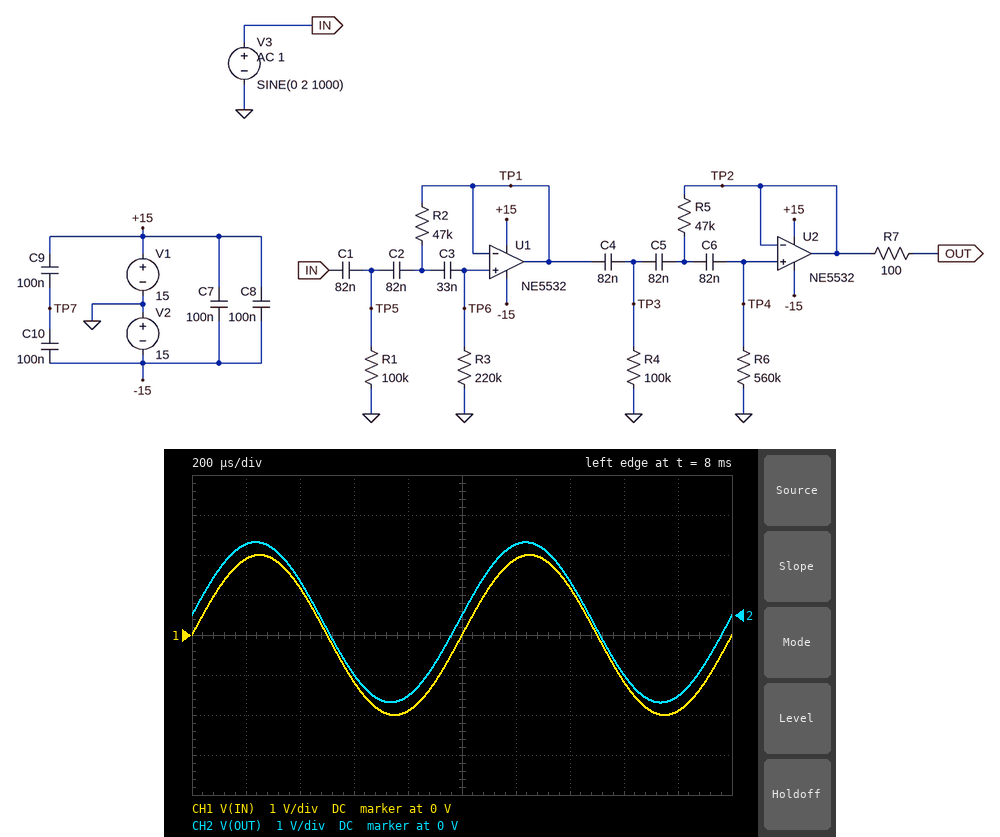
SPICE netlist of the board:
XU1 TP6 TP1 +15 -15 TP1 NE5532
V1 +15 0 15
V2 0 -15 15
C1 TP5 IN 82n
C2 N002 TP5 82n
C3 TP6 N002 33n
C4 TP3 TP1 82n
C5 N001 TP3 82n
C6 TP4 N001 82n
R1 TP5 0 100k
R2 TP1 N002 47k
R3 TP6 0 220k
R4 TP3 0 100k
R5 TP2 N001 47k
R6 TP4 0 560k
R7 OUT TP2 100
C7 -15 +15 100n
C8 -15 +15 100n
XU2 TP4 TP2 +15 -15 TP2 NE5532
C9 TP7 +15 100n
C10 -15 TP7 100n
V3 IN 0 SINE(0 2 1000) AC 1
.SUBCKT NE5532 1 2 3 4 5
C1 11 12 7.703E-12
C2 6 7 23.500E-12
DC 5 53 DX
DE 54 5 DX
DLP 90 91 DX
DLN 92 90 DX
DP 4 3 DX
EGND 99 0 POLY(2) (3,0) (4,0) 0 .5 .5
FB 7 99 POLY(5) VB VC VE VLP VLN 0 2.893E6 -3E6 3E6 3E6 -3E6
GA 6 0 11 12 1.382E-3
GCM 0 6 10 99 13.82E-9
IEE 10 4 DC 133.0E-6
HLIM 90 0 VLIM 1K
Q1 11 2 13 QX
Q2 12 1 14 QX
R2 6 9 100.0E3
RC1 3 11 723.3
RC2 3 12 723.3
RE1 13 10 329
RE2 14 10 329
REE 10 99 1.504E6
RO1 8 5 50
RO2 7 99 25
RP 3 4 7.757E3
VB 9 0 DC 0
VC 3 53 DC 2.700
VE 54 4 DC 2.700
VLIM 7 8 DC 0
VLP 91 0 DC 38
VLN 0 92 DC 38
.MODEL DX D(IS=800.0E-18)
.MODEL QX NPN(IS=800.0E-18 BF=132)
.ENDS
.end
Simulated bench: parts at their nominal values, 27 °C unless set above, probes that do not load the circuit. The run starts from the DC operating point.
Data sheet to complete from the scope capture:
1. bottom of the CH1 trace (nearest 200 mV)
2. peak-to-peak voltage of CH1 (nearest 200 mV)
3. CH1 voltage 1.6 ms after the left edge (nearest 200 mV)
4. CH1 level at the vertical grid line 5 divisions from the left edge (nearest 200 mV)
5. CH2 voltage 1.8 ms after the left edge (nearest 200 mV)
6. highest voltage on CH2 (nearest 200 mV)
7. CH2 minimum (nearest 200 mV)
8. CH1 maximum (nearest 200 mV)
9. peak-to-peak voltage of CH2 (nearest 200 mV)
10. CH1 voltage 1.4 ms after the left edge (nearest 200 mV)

-2.0 V
4.0 V
-1.2 V
0 V
-2.0 V
1.8 V
-2.2 V
2.0 V
4.0 V
1.2 V
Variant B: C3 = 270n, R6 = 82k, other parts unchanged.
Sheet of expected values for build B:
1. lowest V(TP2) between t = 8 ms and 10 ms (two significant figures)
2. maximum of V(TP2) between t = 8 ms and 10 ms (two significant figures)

-2.0 V
2.0 V
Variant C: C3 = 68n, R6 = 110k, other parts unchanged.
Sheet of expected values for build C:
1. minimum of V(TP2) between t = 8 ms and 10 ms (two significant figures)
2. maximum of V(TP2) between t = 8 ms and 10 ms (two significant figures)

-2.0 V
2.0 V
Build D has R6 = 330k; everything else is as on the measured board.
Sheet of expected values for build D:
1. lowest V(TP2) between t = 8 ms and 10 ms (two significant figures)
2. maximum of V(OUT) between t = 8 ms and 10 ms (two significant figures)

-2.1 V
1.9 V
